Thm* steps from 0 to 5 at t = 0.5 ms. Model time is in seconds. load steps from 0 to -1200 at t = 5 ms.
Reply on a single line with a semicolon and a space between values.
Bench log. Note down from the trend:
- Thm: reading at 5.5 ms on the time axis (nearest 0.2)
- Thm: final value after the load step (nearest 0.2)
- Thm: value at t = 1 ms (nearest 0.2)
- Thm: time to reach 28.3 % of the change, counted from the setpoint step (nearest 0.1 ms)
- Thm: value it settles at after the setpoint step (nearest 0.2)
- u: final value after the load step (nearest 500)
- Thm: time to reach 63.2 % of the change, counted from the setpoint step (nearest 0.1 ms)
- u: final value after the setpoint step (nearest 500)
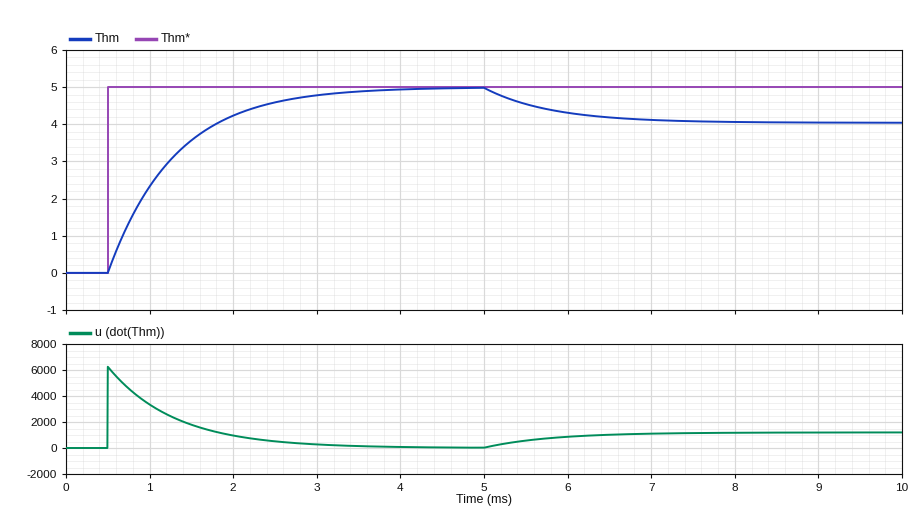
4.6; 4.0; 2.4; 0.3 ms; 5.0; 1000; 0.8 ms; 0
